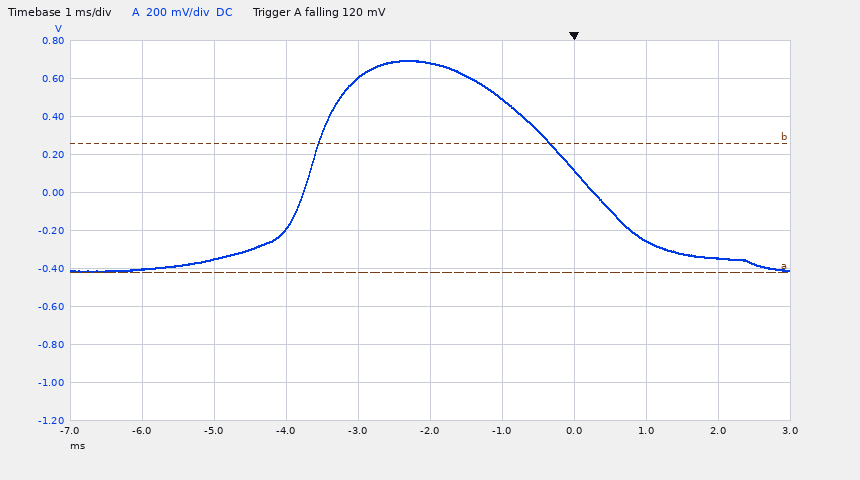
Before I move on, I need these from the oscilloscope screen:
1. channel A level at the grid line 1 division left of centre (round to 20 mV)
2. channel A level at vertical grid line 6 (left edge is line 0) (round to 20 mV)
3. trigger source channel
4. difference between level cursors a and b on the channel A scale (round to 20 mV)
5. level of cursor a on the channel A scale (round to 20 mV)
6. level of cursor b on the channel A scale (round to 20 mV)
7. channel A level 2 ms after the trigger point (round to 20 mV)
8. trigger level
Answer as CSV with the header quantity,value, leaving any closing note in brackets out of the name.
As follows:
quantity,value
channel A level at the grid line 1 division left of centre,600 mV
channel A level at vertical grid line 6 (left edge is line 0),500 mV
trigger source channel,channel A
difference between level cursors a and b on the channel A scale,680 mV
level of cursor a on the channel A scale,-420 mV
level of cursor b on the channel A scale,260 mV
channel A level 2 ms after the trigger point,-340 mV
trigger level,120 mV
